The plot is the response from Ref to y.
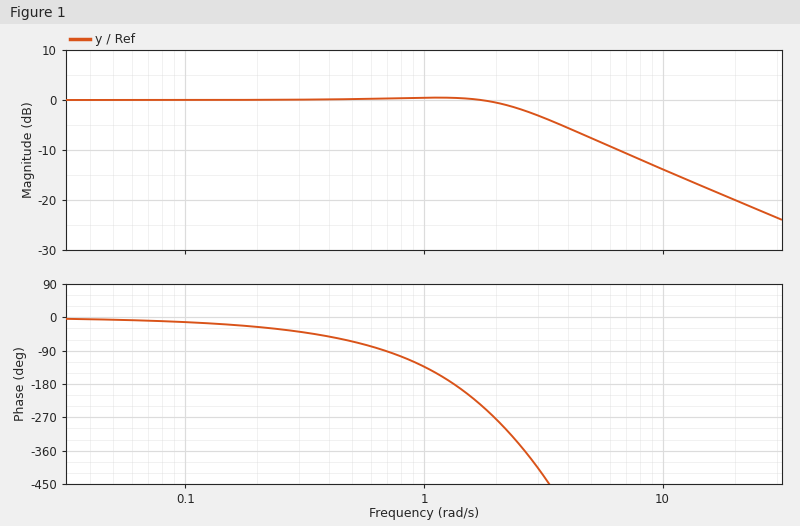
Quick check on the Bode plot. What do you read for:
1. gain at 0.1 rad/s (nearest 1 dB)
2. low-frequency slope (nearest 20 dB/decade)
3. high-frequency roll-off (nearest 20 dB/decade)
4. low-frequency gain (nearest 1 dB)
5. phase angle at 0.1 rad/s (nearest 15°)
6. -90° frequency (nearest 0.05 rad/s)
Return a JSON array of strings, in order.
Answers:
["0 dB", "0 dB/decade", "-20 dB/decade", "0 dB", "-15°", "0.70 rad/s"]
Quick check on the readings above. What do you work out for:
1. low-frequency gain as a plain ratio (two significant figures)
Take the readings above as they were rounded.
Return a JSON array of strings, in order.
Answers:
["1.0"]
